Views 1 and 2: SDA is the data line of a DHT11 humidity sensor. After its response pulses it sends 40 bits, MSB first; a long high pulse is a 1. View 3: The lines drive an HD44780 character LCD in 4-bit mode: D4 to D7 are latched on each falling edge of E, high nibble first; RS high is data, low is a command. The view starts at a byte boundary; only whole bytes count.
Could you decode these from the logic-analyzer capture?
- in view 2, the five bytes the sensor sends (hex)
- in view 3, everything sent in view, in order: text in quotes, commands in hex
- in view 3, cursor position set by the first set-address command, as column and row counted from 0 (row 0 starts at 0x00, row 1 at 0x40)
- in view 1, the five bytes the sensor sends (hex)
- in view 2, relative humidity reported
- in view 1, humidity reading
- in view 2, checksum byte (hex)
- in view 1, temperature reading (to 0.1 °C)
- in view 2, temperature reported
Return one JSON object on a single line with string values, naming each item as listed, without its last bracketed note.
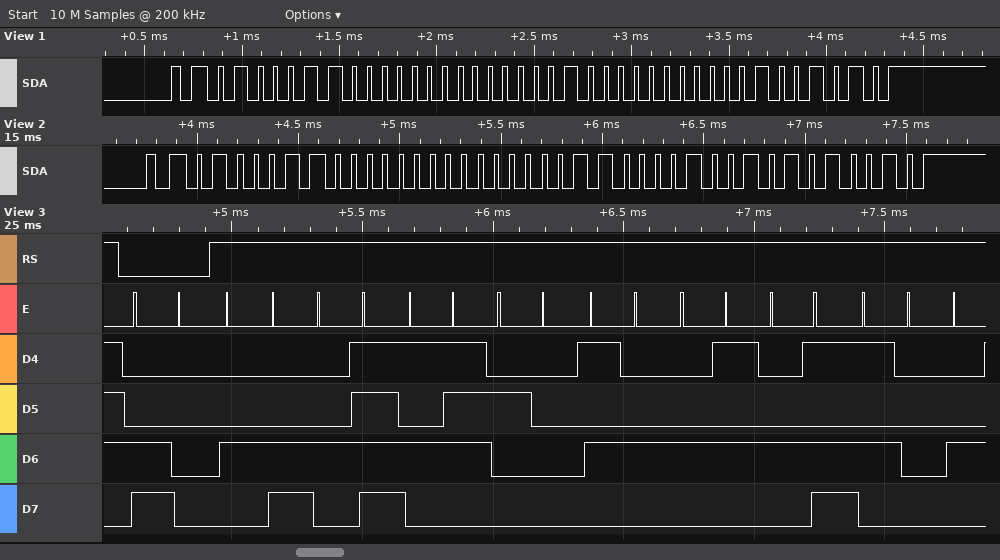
{"in view 2, the five bytes the sensor sends": "46 00 03 09 52", "in view 3, everything sent in view, in order: text in quotes, commands in hex": "0xC0 \"LOW TEMP\"", "in view 3, cursor position set by the first set-address command, as column and row counted from 0": "column 0, row 1", "in view 1, the five bytes the sensor sends": "46 00 04 00 4A", "in view 2, relative humidity reported": "70 %", "in view 1, humidity reading": "70 %", "in view 2, checksum byte": "0x52", "in view 1, temperature reading": "4.0 °C", "in view 2, temperature reported": "3.9 °C"}
